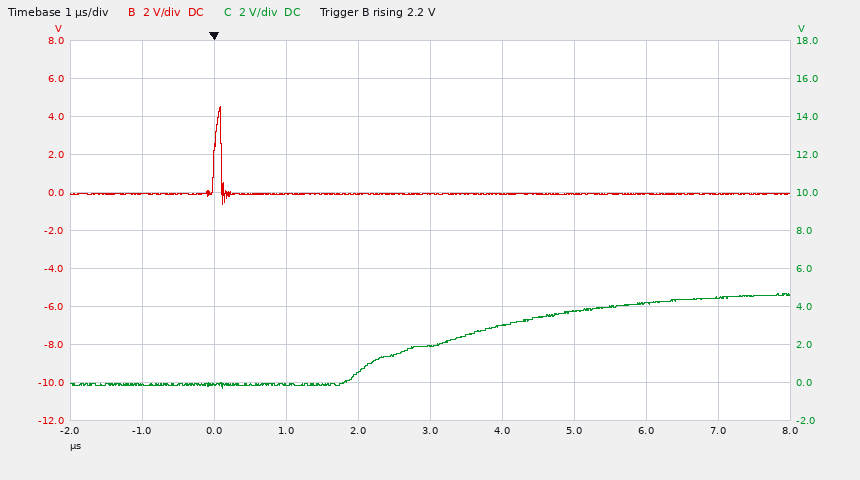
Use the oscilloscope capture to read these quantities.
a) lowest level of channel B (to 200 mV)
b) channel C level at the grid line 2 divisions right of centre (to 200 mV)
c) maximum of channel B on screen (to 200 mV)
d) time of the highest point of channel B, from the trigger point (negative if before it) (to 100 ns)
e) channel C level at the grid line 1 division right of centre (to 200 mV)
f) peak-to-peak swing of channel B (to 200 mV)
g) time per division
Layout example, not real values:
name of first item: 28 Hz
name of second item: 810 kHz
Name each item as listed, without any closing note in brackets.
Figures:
lowest level of channel B: -600 mV
channel C level at the grid line 2 divisions right of centre: 3.8 V
maximum of channel B on screen: 4.6 V
time of the highest point of channel B, from the trigger point (negative if before it): +100 ns
channel C level at the grid line 1 division right of centre: 3.0 V
peak-to-peak swing of channel B: 5.2 V
time per division: 1 µs
